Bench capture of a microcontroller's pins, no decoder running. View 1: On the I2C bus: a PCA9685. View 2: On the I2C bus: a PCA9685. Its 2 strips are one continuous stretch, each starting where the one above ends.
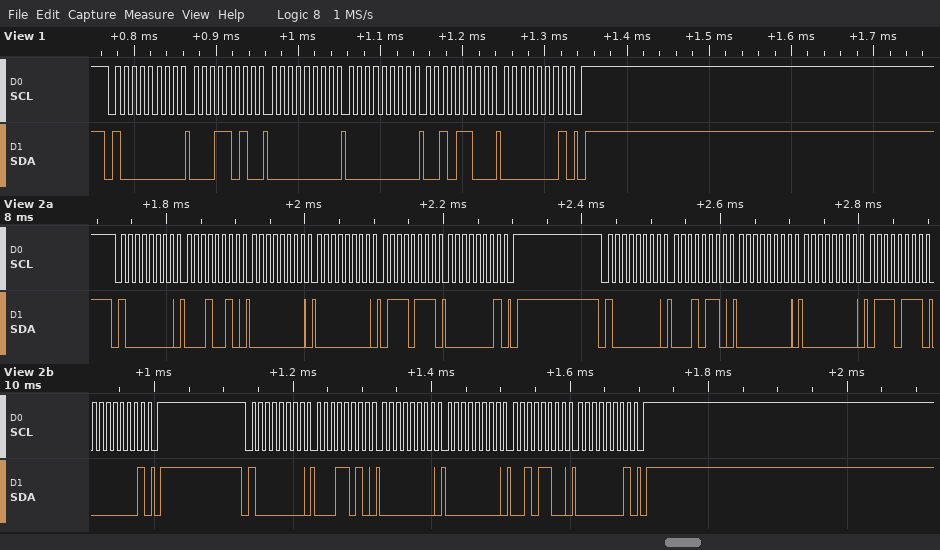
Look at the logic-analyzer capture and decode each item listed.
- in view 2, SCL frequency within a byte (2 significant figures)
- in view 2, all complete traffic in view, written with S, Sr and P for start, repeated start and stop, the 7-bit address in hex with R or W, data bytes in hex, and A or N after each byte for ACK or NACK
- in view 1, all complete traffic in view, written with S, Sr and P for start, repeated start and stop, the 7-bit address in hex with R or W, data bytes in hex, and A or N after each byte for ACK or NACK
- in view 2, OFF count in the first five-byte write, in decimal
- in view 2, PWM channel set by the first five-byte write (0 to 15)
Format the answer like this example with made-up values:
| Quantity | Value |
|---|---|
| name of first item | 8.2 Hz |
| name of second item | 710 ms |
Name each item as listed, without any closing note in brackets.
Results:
| Quantity | Value |
|---|---|
| in view 2, SCL frequency within a byte | 100 kHz |
| in view 2, all complete traffic in view, written with S, Sr and P for start, repeated start and stop, the 7-bit address in hex with R or W, data bytes in hex, and A or N after each byte for ACK or NACK | S 40W A 12 A 00 A 00 A 77 A 01 A P S 40W A 16 A 00 A 00 A 77 A 01 A P S 40W A 1A A 00 A 00 A 2C A 01 A P |
| in view 1, all complete traffic in view, written with S, Sr and P for start, repeated start and stop, the 7-bit address in hex with R or W, data bytes in hex, and A or N after each byte for ACK or NACK | S 40W A 1A A 00 A 00 A 2C A 01 A P |
| in view 2, OFF count in the first five-byte write, in decimal | 375 |
| in view 2, PWM channel set by the first five-byte write | 3 |
